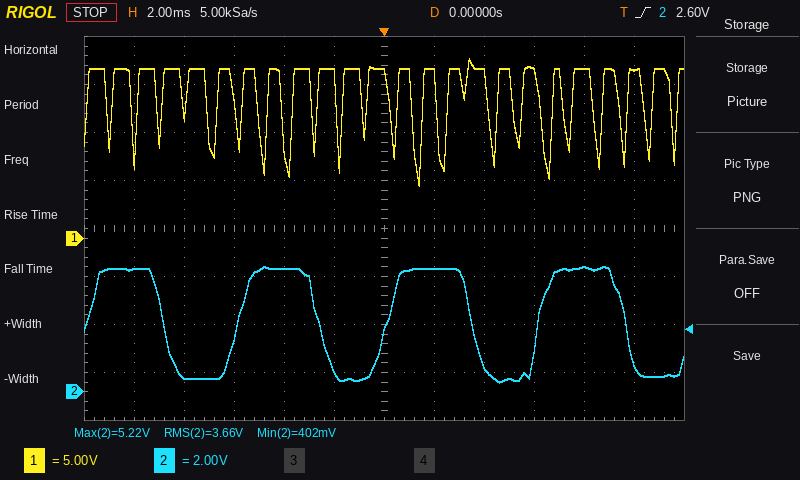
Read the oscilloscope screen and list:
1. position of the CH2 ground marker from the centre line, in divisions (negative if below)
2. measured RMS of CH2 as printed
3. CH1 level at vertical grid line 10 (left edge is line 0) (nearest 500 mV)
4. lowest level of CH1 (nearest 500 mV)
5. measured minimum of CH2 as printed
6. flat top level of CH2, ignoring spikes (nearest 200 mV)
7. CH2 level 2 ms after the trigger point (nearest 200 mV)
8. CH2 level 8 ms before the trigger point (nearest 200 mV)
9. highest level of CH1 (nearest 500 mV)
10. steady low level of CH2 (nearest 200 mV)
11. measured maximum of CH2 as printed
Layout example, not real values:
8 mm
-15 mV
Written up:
-3.4 div
3.66 V
17.5 V
5.5 V
402 mV
5.2 V
5.2 V
600 mV
18.5 V
600 mV
5.22 V
